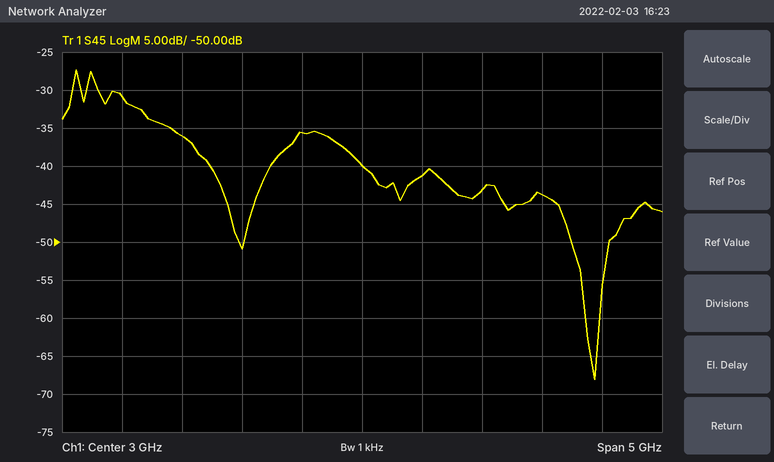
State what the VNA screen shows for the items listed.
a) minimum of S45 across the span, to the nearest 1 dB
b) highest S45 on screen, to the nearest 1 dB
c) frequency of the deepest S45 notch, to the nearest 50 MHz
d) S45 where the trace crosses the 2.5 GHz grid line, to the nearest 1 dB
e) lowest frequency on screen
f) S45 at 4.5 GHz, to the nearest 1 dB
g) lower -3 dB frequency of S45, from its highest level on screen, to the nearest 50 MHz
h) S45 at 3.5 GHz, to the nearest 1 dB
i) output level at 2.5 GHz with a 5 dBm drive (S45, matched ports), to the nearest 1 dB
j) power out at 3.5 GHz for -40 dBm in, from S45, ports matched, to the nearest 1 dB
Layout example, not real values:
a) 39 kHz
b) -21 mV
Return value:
a) -68 dB
b) -27 dB
c) 4.95 GHz
d) -36 dB
e) 500 MHz
f) -44 dB
g) 600 MHz
h) -41 dB
i) -31 dBm
j) -81 dBm
